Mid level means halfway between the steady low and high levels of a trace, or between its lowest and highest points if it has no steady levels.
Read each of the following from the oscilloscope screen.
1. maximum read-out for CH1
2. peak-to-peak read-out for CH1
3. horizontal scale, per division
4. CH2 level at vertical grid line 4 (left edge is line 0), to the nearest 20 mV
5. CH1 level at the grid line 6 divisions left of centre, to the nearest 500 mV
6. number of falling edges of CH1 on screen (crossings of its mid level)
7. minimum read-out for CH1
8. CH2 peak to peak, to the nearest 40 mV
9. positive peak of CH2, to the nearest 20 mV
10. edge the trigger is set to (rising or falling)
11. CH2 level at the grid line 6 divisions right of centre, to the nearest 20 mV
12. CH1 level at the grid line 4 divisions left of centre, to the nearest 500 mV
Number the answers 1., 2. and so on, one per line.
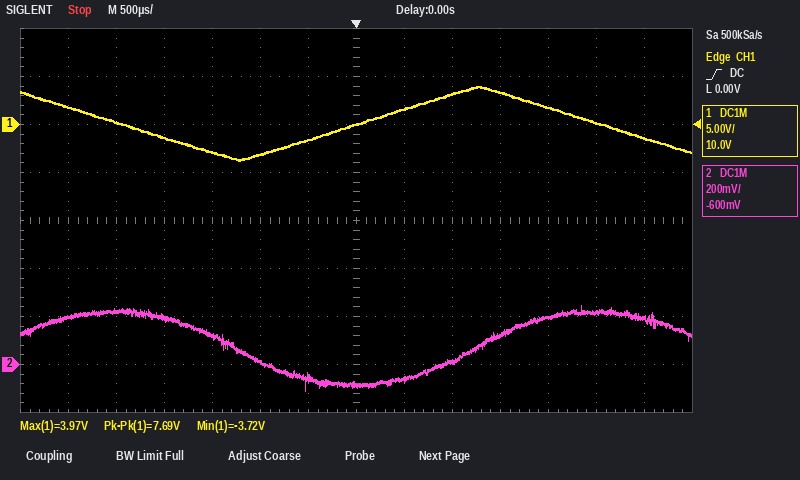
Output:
1. 3.97 V
2. 7.69 V
3. 500 µs
4. 120 mV
5. 2.0 V
6. 2
7. -3.72 V
8. 360 mV
9. 240 mV
10. rising
11. 200 mV
12. -1.5 V
